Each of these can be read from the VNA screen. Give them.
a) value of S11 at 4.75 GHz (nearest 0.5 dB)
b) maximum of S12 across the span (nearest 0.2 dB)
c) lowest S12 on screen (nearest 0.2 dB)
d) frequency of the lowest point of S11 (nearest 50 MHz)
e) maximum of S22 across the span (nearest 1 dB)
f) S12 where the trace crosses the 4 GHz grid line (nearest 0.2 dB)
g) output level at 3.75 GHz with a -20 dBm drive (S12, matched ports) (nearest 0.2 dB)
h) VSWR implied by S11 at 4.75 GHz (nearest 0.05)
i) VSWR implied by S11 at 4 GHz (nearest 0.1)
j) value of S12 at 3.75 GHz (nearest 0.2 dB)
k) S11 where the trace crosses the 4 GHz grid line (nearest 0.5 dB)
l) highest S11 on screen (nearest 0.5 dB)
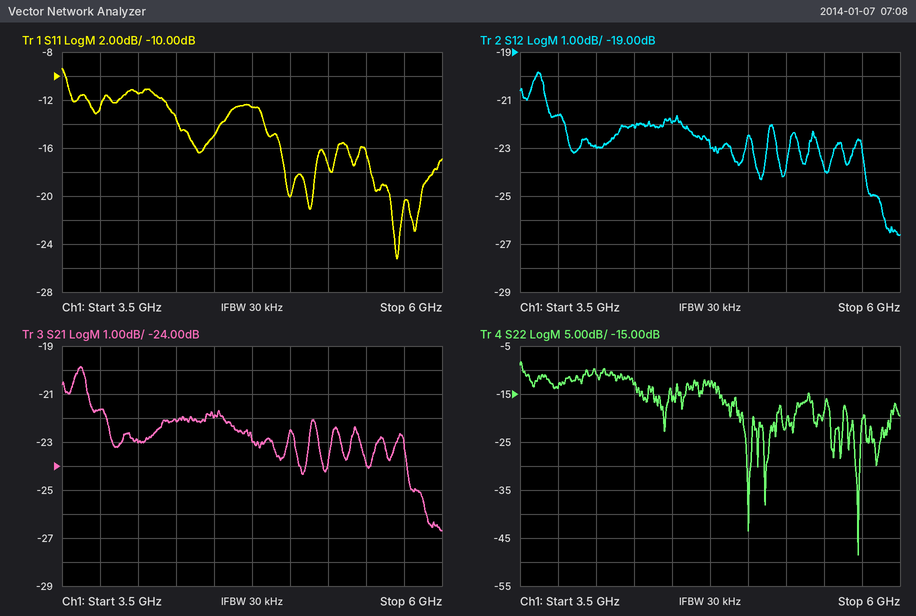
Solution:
-12.5 dB
-19.8 dB
-26.6 dB
5.70 GHz
-8 dB
-23.0 dB
-41.6 dBm
1.60
1.7
-21.6 dB
-11.5 dB
-9.5 dB
